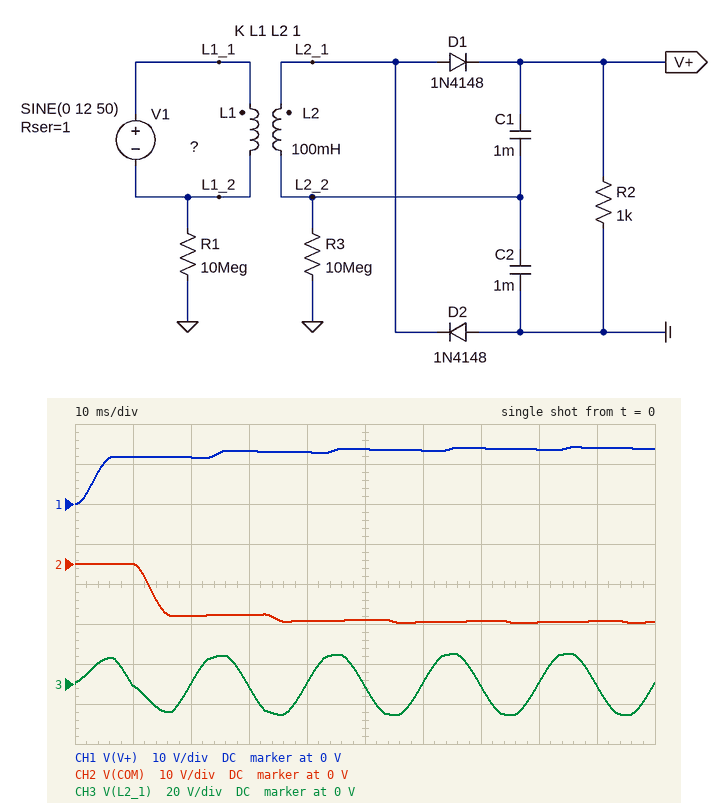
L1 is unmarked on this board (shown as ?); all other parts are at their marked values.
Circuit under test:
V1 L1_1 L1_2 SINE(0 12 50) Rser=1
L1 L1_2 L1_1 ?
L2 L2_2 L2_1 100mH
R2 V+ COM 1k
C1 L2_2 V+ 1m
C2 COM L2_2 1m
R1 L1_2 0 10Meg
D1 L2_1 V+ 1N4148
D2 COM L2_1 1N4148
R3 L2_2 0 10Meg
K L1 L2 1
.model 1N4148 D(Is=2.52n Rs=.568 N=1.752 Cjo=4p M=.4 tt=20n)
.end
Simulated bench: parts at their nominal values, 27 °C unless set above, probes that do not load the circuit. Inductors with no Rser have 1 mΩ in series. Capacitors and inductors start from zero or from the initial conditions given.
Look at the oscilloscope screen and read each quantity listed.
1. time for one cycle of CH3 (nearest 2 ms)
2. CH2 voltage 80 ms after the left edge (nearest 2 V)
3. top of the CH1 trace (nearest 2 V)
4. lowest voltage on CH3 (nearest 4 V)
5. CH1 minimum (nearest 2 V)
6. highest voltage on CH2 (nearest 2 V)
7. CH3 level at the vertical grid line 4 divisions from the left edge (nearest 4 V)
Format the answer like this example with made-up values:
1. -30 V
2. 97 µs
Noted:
1. 20 ms
2. -14 V
3. 14 V
4. -16 V
5. 0 V
6. 0 V
7. 0 V
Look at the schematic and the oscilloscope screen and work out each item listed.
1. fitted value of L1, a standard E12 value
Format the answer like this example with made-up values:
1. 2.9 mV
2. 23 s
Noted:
1. 56 mH
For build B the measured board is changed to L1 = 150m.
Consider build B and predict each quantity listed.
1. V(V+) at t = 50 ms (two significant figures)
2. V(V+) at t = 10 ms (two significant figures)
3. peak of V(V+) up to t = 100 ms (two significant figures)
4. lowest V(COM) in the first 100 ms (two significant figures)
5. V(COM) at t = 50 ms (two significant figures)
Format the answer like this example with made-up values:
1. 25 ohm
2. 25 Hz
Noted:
1. 8.5 V
2. 8.1 V
3. 8.6 V
4. -8.9 V
5. -8.6 V
